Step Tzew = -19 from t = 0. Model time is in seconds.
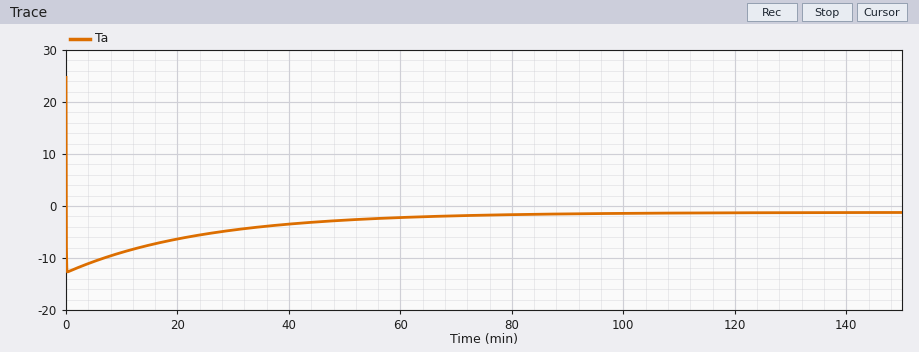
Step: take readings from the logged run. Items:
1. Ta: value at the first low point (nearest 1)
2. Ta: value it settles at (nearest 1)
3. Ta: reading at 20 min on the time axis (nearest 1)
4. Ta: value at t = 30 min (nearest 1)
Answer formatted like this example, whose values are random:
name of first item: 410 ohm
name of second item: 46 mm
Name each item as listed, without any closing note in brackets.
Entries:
Ta: value at the first low point: -13
Ta: value it settles at: -1
Ta: reading at 20 min on the time axis: -6
Ta: value at t = 30 min: -5
